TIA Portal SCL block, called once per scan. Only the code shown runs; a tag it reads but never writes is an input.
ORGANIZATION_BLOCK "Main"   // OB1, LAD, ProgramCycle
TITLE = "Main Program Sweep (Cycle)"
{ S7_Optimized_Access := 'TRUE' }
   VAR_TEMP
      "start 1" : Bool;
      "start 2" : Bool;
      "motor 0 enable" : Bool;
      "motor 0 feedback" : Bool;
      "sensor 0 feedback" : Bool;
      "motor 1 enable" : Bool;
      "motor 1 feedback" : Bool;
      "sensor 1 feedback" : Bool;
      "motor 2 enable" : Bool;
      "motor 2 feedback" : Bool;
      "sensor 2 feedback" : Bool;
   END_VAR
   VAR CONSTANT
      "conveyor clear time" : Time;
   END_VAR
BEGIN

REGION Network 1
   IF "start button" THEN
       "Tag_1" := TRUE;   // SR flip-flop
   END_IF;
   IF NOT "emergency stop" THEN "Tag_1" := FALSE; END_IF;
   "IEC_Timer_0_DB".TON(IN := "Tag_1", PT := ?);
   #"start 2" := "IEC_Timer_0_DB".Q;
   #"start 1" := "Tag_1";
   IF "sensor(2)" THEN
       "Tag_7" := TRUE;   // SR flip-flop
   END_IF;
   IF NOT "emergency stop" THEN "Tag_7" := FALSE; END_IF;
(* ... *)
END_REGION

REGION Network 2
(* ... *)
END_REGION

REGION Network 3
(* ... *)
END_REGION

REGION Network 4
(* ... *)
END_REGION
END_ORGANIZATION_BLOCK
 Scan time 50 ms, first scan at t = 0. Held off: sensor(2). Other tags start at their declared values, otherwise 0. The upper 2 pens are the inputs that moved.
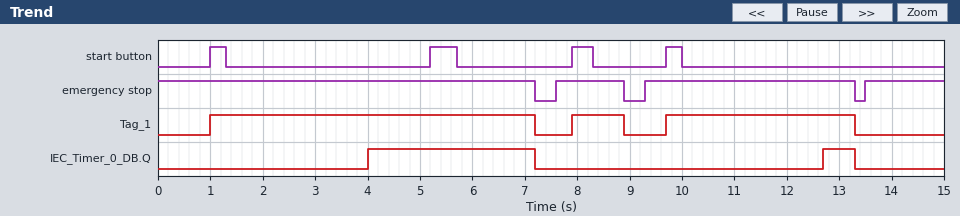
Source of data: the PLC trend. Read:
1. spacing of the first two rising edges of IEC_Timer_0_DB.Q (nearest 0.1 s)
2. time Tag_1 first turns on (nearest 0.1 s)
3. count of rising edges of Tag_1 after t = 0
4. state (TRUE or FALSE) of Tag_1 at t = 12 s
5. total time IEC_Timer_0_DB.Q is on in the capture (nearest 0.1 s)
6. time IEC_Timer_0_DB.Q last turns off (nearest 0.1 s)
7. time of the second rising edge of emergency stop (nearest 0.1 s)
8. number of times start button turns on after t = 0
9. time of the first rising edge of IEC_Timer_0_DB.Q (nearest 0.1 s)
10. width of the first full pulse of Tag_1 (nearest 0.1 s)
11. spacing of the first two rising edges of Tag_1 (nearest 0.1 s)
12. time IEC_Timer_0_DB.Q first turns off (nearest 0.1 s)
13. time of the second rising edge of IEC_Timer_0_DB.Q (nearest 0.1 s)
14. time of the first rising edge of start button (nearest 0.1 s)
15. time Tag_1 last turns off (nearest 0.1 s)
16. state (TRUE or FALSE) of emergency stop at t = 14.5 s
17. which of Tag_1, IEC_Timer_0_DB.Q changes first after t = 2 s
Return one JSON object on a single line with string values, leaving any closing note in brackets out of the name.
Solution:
{"spacing of the first two rising edges of IEC_Timer_0_DB.Q": "8.7 s", "time Tag_1 first turns on": "1.0 s", "count of rising edges of Tag_1 after t = 0": "3", "state (TRUE or FALSE) of Tag_1 at t = 12 s": "TRUE", "total time IEC_Timer_0_DB.Q is on in the capture": "3.8 s", "time IEC_Timer_0_DB.Q last turns off": "13.3 s", "time of the second rising edge of emergency stop": "9.3 s", "number of times start button turns on after t = 0": "4", "time of the first rising edge of IEC_Timer_0_DB.Q": "4.0 s", "width of the first full pulse of Tag_1": "6.2 s", "spacing of the first two rising edges of Tag_1": "6.9 s", "time IEC_Timer_0_DB.Q first turns off": "7.2 s", "time of the second rising edge of IEC_Timer_0_DB.Q": "12.7 s", "time of the first rising edge of start button": "1.0 s", "time Tag_1 last turns off": "13.3 s", "state (TRUE or FALSE) of emergency stop at t = 14.5 s": "TRUE", "which of Tag_1, IEC_Timer_0_DB.Q changes first after t = 2 s": "IEC_Timer_0_DB.Q"}
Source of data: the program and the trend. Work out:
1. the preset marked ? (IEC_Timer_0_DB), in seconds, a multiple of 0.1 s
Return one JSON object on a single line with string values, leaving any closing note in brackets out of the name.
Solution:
{"the preset marked ? (IEC_Timer_0_DB), in seconds, a multiple of 0.1 s": "3.0 s"}
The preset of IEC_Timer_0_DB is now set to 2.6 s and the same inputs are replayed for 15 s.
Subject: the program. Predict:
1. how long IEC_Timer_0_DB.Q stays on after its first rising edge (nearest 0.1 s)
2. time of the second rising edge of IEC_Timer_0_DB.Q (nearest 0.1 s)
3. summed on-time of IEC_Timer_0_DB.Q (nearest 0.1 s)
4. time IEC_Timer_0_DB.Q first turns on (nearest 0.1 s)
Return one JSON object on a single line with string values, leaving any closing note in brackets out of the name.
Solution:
{"how long IEC_Timer_0_DB.Q stays on after its first rising edge": "3.6 s", "time of the second rising edge of IEC_Timer_0_DB.Q": "12.3 s", "summed on-time of IEC_Timer_0_DB.Q": "4.6 s", "time IEC_Timer_0_DB.Q first turns on": "3.6 s"}
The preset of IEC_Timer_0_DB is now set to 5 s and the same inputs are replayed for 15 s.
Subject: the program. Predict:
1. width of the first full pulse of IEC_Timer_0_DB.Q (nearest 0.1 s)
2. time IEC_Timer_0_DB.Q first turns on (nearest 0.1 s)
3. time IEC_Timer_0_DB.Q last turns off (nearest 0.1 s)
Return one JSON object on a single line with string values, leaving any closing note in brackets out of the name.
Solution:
{"width of the first full pulse of IEC_Timer_0_DB.Q": "1.2 s", "time IEC_Timer_0_DB.Q first turns on": "6.0 s", "time IEC_Timer_0_DB.Q last turns off": "7.2 s"}
